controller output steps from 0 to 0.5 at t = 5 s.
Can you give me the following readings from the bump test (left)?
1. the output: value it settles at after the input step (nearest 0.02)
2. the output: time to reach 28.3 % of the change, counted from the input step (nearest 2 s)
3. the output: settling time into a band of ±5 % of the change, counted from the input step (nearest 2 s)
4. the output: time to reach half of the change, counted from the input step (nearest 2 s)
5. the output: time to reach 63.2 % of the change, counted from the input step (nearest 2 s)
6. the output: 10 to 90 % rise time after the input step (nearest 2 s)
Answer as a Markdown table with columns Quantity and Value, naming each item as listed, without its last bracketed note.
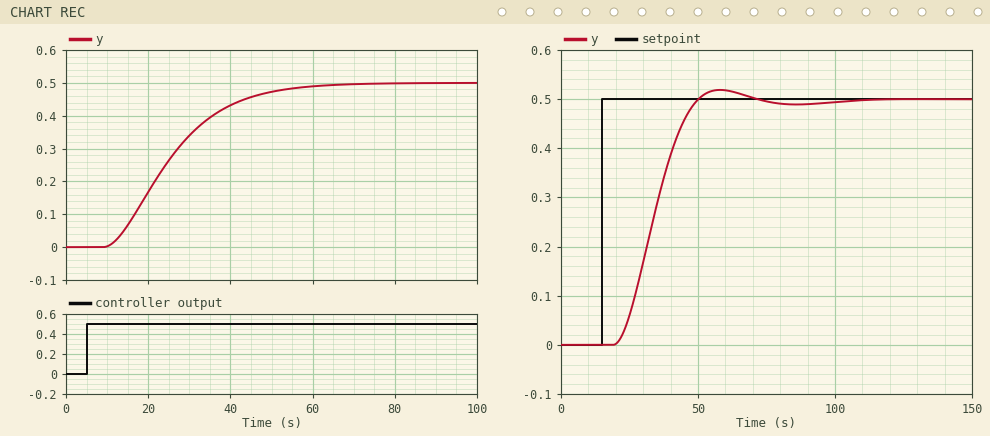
| Quantity | Value |
|---|---|
| the output: value it settles at after the input step | 0.50 |
| the output: time to reach 28.3 % of the change, counted from the input step | 14 s |
| the output: settling time into a band of ±5 % of the change, counted from the input step | 46 s |
| the output: time to reach half of the change, counted from the input step | 20 s |
| the output: time to reach 63.2 % of the change, counted from the input step | 24 s |
| the output: 10 to 90 % rise time after the input step | 30 s |
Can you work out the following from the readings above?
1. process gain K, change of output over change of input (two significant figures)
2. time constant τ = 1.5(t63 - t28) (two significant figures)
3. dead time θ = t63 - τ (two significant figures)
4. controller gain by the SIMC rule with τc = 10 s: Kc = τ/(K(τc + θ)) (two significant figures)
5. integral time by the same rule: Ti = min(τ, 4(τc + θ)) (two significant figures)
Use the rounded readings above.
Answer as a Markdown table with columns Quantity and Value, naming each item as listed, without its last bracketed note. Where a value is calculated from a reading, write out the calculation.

| Quantity | Value |
|---|---|
| process gain K, change of output over change of input | (0.5 - 0) / 0.5 = 1.0 |
| time constant τ = 1.5(t63 - t28) | 1.5 × (24 - 14) = 15 s |
| dead time θ = t63 - τ | 24 - 15 = 9.0 s |
| controller gain by the SIMC rule with τc = 10 s: Kc = τ/(K(τc + θ)) | 15 / (1 × (10 + 9)) = 0.79 |
| integral time by the same rule: Ti = min(τ, 4(τc + θ)) | min(15, 4 × (10 + 9)) = 15 s |
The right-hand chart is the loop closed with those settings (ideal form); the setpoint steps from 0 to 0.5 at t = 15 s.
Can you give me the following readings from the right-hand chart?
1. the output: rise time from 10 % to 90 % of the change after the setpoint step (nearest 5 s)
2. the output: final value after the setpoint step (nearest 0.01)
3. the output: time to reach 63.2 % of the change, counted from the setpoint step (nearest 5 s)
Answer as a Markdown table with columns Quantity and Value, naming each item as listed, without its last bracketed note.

| Quantity | Value |
|---|---|
| the output: rise time from 10 % to 90 % of the change after the setpoint step | 20 s |
| the output: final value after the setpoint step | 0.50 |
| the output: time to reach 63.2 % of the change, counted from the setpoint step | 20 s |
